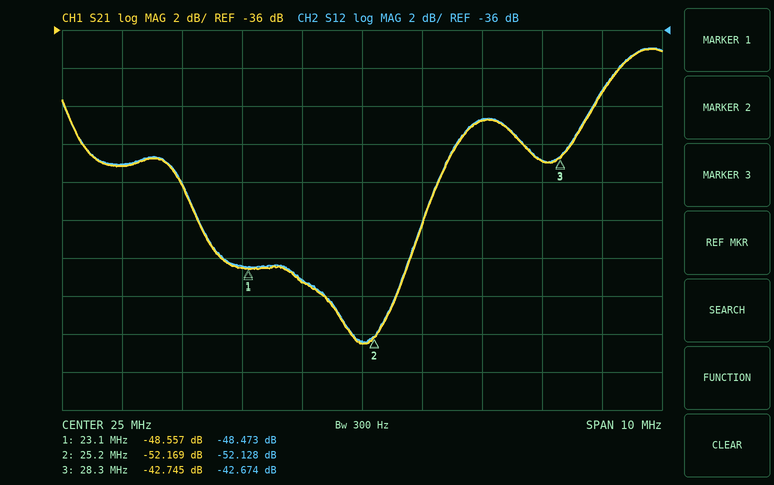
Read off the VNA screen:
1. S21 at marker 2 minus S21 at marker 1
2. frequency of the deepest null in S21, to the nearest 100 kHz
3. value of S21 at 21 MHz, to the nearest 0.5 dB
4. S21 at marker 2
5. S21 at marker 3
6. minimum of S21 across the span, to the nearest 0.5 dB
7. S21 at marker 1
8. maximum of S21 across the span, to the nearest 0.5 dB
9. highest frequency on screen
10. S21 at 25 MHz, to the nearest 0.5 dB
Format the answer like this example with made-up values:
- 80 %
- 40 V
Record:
- -3.612 dB
- 25.0 MHz
- -43.0 dB
- -52.169 dB
- -42.745 dB
- -52.5 dB
- -48.557 dB
- -37.0 dB
- 30 MHz
- -52.5 dB
